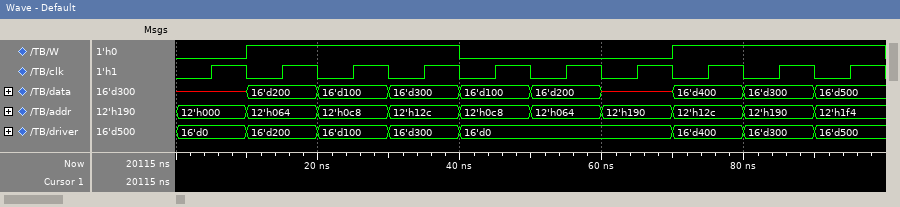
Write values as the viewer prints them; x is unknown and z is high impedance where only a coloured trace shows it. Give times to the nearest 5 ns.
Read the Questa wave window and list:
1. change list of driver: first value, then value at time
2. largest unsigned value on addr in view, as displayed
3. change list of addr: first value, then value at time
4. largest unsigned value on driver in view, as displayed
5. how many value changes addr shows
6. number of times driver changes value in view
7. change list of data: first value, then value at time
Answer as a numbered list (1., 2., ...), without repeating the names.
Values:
1. 16'd0, 16'd200 at 10 ns, 16'd100 at 20 ns, 16'd300 at 30 ns, 16'd0 at 40 ns, 16'd400 at 70 ns, 16'd300 at 80 ns, 16'd500 at 90 ns
2. 12'h1f4
3. 12'h000, 12'h064 at 10 ns, 12'h0c8 at 20 ns, 12'h12c at 30 ns, 12'h0c8 at 40 ns, 12'h064 at 50 ns, 12'h190 at 60 ns, 12'h12c at 70 ns, 12'h190 at 80 ns, 12'h1f4 at 90 ns
4. 16'd500
5. 9
6. 7
7. x, 16'd200 at 10 ns, 16'd100 at 20 ns, 16'd300 at 30 ns, 16'd100 at 40 ns, 16'd200 at 50 ns, x at 60 ns, 16'd400 at 70 ns, 16'd300 at 80 ns, 16'd500 at 90 ns
